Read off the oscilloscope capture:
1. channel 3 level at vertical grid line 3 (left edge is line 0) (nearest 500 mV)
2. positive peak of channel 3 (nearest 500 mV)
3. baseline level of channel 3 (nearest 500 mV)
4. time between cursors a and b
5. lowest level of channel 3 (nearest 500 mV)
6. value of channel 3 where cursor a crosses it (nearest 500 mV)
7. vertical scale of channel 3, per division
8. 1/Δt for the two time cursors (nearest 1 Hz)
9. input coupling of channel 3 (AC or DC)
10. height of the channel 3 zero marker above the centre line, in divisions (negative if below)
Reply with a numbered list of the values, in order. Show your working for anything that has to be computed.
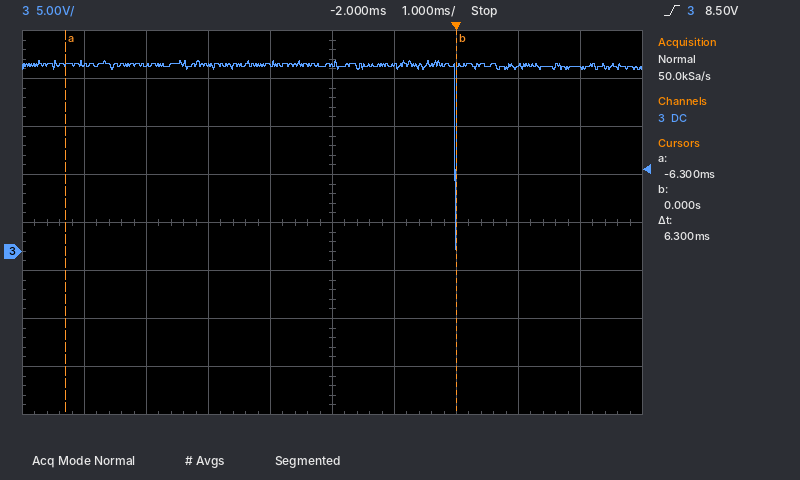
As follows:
1. 19.5 V
2. 20.0 V
3. 19.5 V
4. 6.3 ms
5. 0.0 V
6. 19.5 V
7. 5 V
8. 1 / 6.3 ms ≈ 159 Hz
9. DC
10. -0.6 div
